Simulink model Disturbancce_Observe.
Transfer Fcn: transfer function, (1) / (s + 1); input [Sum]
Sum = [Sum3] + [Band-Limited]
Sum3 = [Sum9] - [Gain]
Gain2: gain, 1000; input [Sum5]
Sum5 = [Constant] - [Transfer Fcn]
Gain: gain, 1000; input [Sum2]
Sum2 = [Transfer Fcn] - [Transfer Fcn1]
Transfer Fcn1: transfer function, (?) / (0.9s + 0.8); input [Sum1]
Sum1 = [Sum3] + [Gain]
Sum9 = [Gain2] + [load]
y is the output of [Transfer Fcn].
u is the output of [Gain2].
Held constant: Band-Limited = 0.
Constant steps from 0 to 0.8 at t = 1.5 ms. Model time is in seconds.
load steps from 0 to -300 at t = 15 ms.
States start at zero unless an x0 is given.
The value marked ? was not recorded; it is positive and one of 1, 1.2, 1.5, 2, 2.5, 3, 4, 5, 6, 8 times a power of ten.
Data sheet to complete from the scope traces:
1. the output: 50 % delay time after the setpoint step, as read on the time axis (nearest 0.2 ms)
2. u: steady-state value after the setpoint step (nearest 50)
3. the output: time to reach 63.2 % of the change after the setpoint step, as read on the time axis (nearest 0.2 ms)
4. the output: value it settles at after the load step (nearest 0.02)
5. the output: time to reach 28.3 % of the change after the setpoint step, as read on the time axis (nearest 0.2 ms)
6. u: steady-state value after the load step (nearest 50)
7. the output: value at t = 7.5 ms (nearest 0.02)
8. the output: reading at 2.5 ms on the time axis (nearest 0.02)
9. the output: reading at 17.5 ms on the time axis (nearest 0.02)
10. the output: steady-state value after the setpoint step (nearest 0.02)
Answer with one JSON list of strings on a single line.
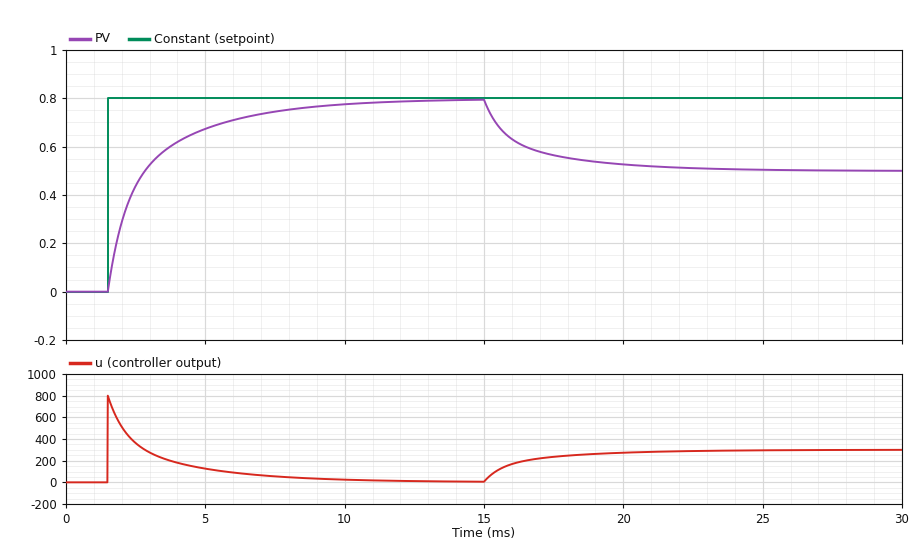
["2.4 ms", "0", "2.8 ms", "0.50", "1.8 ms", "300", "0.74", "0.44", "0.56", "0.80"]
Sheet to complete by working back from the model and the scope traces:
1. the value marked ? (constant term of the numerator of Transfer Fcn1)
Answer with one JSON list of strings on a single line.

["0.5"]
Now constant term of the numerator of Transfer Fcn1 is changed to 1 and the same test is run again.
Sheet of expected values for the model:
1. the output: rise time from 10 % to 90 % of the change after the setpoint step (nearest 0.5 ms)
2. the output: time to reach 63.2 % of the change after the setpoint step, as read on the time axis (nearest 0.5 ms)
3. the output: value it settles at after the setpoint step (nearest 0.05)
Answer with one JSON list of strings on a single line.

["2.0 ms", "2.5 ms", "0.80"]
